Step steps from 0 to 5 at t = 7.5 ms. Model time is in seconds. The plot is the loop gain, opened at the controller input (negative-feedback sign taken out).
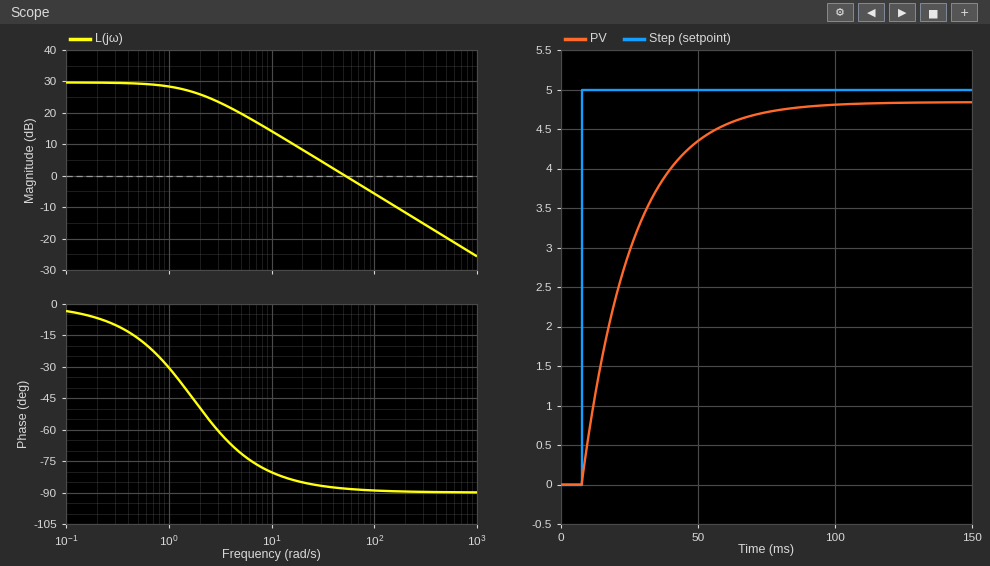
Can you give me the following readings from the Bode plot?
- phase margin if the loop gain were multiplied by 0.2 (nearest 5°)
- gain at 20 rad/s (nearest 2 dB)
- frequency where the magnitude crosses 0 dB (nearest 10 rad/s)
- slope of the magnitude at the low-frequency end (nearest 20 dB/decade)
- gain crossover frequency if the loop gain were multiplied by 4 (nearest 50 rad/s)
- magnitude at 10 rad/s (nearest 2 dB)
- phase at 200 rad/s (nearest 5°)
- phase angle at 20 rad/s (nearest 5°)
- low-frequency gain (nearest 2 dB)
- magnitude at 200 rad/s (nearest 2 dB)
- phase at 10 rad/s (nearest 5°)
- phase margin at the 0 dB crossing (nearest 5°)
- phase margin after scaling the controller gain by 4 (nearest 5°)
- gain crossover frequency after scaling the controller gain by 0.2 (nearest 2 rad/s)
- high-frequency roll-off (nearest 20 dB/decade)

100°
8 dB
50 rad/s
0 dB/decade
200 rad/s
14 dB
-90°
-85°
30 dB
-12 dB
-80°
90°
90°
10 rad/s
-20 dB/decade
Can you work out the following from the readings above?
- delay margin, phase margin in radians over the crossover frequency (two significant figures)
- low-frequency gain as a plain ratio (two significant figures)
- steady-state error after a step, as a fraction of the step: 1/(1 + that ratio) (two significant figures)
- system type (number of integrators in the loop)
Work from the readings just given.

0.031 s
32
0.030
0
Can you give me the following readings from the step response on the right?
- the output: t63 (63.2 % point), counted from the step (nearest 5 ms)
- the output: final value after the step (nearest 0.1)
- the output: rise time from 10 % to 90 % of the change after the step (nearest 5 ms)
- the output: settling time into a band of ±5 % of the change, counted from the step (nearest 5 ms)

20 ms
4.8
40 ms
55 ms
